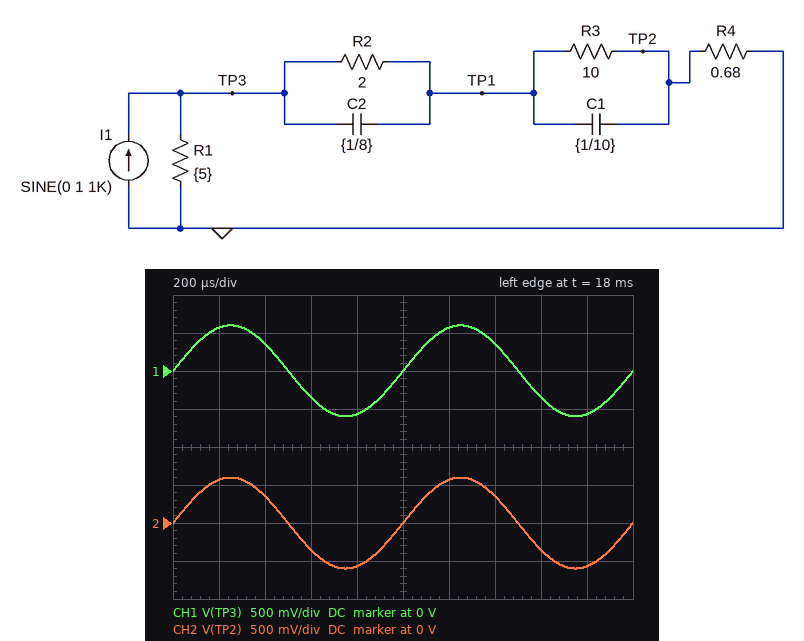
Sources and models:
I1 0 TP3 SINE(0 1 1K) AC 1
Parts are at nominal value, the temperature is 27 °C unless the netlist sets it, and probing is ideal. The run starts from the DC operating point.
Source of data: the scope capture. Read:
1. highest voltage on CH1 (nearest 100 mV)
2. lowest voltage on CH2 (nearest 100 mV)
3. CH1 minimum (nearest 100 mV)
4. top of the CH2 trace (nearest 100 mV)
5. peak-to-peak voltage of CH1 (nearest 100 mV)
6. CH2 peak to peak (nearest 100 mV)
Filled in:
600 mV
-600 mV
-600 mV
600 mV
1.2 V
1.2 V
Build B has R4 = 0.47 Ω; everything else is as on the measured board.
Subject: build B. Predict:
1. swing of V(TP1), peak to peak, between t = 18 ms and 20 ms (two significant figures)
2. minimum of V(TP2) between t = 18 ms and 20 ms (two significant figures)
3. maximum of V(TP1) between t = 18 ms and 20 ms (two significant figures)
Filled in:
860 mV
-430 mV
430 mV
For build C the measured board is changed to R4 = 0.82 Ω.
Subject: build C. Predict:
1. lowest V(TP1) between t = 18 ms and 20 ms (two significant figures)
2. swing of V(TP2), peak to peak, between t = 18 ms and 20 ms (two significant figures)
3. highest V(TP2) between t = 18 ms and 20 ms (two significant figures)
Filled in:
-700 mV
1.4 V
700 mV
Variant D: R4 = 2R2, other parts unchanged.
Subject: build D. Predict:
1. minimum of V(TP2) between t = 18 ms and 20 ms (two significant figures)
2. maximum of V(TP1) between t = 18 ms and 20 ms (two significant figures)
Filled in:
-1.5 V
1.5 V
